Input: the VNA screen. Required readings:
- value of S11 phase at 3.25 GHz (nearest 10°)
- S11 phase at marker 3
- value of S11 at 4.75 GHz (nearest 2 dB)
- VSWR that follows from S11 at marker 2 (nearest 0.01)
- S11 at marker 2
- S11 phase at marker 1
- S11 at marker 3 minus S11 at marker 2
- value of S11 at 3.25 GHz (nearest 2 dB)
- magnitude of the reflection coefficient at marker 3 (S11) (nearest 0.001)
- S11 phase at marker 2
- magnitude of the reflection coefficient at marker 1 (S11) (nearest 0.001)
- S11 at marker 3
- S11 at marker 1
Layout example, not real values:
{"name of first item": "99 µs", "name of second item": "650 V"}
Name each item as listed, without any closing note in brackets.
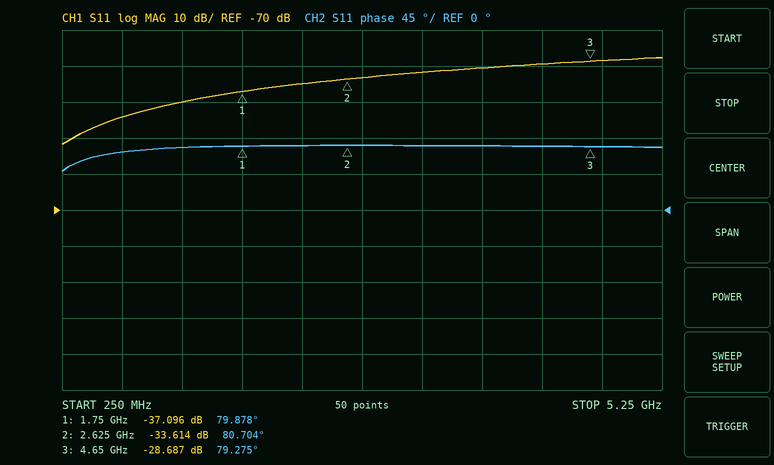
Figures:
{"value of S11 phase at 3.25 GHz": "80°", "S11 phase at marker 3": "79.275°", "value of S11 at 4.75 GHz": "-28 dB", "VSWR that follows from S11 at marker 2": "1.04", "S11 at marker 2": "-33.614 dB", "S11 phase at marker 1": "79.878°", "S11 at marker 3 minus S11 at marker 2": "4.927 dB", "value of S11 at 3.25 GHz": "-32 dB", "magnitude of the reflection coefficient at marker 3 (S11)": "0.037", "S11 phase at marker 2": "80.704°", "magnitude of the reflection coefficient at marker 1 (S11)": "0.014", "S11 at marker 3": "-28.687 dB", "S11 at marker 1": "-37.096 dB"}
